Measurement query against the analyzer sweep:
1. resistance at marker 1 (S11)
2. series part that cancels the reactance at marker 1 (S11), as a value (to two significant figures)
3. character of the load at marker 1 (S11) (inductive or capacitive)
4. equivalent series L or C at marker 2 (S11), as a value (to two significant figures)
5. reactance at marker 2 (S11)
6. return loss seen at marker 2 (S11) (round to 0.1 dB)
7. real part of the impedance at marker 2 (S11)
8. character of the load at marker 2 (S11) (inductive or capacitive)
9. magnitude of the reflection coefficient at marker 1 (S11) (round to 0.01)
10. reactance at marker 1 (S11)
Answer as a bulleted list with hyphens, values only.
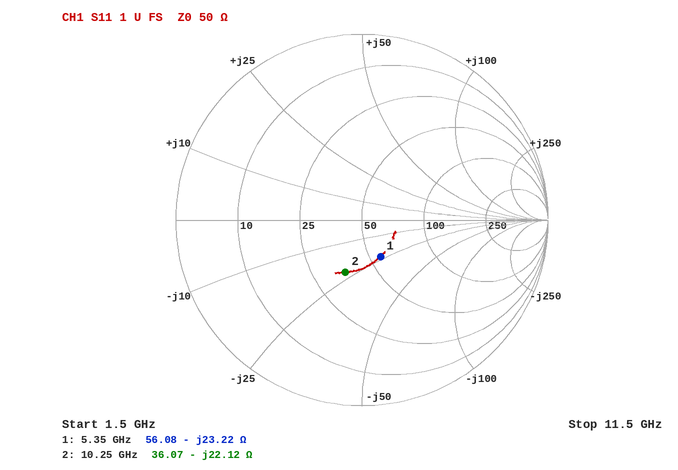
- 56.08 Ω
- 690 pH
- capacitive
- 700 fF
- -22.12 Ω
- 10.6 dB
- 36.07 Ω
- capacitive
- 0.22
- -23.22 Ω
